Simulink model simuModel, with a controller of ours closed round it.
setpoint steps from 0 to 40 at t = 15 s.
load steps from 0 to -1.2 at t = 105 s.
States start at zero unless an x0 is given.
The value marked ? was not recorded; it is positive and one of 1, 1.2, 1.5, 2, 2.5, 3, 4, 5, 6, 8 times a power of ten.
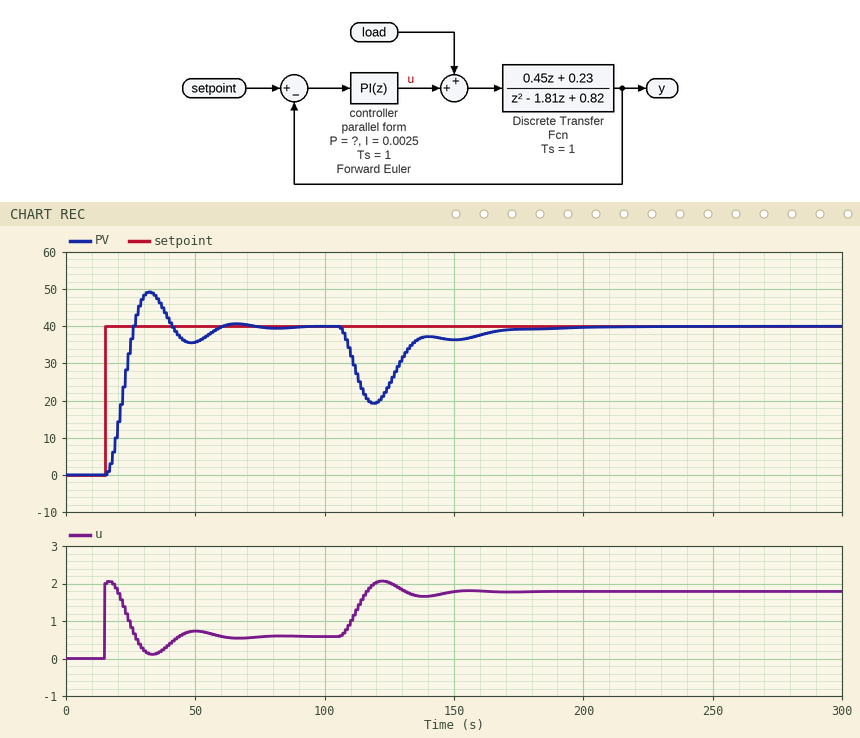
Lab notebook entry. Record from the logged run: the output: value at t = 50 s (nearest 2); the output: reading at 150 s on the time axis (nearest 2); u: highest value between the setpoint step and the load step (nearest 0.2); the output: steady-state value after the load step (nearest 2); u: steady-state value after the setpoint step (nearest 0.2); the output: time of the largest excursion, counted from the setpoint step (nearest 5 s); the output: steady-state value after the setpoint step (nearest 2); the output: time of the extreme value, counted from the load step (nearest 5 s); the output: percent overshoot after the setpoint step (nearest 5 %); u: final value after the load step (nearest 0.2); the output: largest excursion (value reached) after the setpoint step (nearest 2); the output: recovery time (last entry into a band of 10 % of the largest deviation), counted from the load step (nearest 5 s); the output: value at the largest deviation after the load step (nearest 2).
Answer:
36
36
2.0
40
0.6
15 s
40
15 s
25 %
1.8
50
55 s
20
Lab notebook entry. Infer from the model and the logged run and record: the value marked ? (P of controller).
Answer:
0.05
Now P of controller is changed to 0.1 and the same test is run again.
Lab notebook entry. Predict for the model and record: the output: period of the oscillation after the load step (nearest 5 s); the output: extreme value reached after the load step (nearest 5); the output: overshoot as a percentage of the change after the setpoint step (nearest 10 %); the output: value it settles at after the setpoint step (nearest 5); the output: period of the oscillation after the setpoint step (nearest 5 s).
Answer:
20 s
25
30 %
40
25 s
